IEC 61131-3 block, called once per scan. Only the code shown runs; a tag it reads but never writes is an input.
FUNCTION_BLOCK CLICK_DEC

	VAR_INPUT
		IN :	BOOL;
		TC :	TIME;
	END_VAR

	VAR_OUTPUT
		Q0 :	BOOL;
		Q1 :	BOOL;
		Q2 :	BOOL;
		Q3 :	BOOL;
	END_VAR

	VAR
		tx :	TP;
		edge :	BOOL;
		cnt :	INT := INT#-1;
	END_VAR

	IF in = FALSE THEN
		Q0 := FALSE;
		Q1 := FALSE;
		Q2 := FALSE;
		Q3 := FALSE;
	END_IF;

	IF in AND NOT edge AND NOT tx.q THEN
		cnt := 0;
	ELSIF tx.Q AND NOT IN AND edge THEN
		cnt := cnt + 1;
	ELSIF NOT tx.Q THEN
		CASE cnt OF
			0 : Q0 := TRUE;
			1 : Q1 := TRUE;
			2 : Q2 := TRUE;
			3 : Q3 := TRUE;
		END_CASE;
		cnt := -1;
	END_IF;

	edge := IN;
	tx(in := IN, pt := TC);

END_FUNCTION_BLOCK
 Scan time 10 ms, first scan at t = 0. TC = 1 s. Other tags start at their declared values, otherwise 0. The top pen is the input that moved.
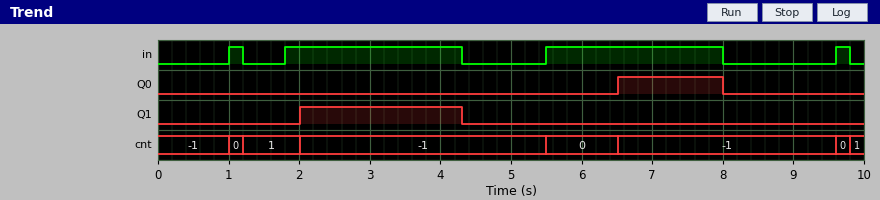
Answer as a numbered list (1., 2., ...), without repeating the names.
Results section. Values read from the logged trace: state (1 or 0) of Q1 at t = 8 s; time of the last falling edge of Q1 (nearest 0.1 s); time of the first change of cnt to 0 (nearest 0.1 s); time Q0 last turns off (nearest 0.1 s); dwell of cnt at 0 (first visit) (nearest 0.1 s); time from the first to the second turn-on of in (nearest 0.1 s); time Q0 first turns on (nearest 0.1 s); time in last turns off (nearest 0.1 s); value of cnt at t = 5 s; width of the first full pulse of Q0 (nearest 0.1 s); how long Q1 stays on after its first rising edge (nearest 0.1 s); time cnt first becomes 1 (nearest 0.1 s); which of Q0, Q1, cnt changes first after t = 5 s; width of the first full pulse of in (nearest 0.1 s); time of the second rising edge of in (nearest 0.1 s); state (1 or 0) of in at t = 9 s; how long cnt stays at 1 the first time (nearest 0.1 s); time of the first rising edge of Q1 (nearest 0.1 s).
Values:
1. 0
2. 4.3 s
3. 1.0 s
4. 8.0 s
5. 0.2 s
6. 0.8 s
7. 6.5 s
8. 9.8 s
9. -1
10. 1.5 s
11. 2.3 s
12. 1.2 s
13. cnt
14. 0.2 s
15. 1.8 s
16. 0
17. 0.8 s
18. 2.0 s
